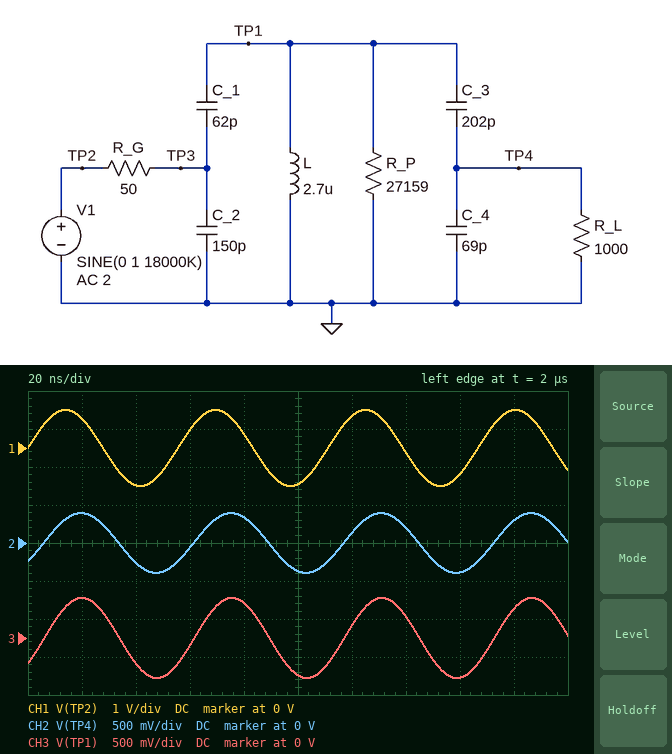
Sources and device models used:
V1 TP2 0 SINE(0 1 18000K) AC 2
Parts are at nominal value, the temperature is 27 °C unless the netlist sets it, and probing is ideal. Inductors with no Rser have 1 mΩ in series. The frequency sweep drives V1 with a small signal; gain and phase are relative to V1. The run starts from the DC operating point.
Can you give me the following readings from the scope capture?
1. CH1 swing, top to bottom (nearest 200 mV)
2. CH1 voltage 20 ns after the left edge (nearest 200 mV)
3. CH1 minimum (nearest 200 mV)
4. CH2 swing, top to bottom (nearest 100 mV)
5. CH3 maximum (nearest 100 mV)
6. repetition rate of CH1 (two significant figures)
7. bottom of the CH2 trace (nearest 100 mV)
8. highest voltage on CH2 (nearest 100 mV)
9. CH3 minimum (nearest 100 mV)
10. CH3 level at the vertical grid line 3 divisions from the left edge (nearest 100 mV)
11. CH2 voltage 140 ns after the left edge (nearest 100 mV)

2.0 V
800 mV
-1.0 V
800 mV
500 mV
18 MHz
-400 mV
400 mV
-500 mV
-100 mV
200 mV
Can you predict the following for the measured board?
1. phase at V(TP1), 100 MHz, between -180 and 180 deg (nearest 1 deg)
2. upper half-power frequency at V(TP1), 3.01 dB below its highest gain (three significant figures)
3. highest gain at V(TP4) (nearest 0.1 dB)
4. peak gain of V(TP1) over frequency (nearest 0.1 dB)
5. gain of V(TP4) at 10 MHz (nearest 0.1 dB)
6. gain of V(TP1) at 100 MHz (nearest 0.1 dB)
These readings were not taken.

-79 deg
10.2 MHz
6.7 dB
9.2 dB
4.5 dB
-20.3 dB
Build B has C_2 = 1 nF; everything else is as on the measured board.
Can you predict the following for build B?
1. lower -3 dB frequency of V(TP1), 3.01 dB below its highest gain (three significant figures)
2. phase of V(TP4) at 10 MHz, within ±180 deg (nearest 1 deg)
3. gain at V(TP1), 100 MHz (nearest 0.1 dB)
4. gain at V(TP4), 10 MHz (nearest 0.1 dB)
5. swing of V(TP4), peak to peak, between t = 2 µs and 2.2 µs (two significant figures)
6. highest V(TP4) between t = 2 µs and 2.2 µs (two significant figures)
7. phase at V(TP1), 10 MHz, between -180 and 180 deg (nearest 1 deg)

8.75 MHz
-38 deg
-35.4 dB
-3.5 dB
190 mV
93 mV
-42 deg
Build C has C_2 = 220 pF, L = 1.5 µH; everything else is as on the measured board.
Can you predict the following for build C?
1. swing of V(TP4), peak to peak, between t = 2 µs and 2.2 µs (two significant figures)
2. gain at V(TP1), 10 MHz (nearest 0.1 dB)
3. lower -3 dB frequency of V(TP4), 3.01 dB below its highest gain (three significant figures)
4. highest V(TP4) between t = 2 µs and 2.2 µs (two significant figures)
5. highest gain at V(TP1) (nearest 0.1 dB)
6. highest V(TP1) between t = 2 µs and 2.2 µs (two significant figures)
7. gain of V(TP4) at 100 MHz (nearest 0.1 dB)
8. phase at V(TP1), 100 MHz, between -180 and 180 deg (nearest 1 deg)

930 mV
-2.7 dB
11.8 MHz
460 mV
9.3 dB
620 mV
-25.6 dB
-82 deg
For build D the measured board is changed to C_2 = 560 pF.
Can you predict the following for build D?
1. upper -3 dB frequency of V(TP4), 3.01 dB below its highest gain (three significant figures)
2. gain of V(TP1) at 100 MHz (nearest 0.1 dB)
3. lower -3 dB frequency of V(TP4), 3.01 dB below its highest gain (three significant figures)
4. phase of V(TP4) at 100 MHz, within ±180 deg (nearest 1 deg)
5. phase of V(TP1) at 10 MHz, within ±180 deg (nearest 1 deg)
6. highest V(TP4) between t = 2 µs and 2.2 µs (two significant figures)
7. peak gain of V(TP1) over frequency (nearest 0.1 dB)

9.84 MHz
-30.5 dB
8.74 MHz
-86 deg
-25 deg
160 mV
7.4 dB
